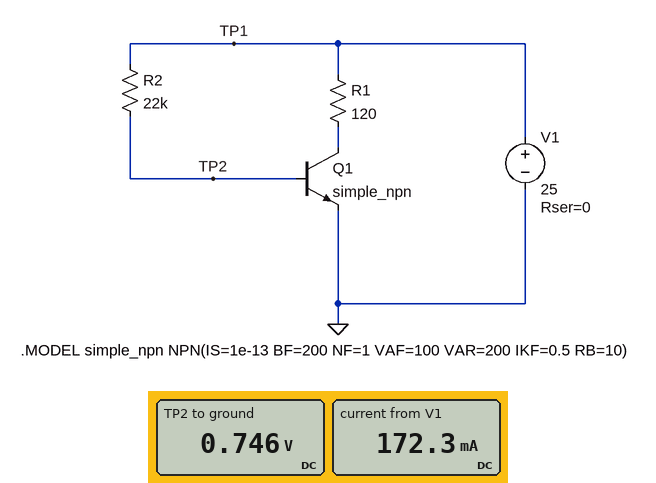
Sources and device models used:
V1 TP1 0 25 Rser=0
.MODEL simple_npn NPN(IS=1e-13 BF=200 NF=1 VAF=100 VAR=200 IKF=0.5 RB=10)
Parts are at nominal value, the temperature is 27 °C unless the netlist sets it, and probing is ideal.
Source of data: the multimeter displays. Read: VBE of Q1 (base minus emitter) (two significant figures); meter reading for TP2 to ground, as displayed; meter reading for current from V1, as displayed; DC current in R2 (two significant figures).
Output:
750 mV
0.746 V
172.3 mA
1.1 mA
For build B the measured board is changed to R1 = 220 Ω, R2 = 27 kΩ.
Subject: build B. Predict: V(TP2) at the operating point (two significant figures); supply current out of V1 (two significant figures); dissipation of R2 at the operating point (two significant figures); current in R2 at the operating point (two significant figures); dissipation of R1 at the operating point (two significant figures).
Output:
730 mV
110 mA
22 mW
900 µA
2.8 W
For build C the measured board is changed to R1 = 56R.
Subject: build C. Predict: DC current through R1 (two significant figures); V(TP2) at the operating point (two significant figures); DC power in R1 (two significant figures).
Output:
190 mA
750 mV
2.0 W
